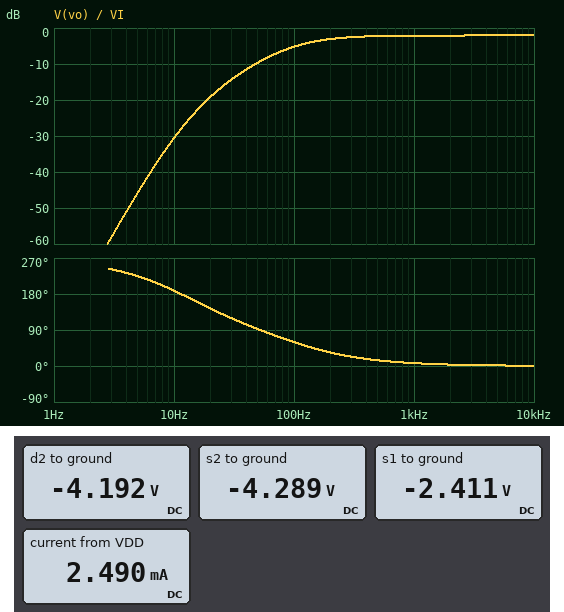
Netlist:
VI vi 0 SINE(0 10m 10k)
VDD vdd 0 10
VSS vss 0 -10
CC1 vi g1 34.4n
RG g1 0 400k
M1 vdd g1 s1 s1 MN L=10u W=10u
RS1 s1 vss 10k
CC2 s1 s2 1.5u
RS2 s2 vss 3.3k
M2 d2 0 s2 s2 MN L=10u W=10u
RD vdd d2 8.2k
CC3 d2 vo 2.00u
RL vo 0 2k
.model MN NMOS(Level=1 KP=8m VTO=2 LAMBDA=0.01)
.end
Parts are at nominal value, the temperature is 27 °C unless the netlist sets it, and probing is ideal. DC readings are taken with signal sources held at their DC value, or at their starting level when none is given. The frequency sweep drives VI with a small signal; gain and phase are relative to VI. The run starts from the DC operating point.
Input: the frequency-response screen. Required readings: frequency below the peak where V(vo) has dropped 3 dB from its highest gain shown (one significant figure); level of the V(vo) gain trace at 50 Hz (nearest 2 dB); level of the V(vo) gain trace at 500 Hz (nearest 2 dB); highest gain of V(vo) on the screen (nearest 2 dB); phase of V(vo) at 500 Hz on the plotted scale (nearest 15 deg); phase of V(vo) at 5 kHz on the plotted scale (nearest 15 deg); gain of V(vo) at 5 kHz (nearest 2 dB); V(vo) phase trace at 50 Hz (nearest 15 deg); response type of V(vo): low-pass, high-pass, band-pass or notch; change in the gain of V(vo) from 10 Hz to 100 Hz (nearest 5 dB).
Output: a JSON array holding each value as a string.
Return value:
["100 Hz", "-10 dB", "-2 dB", "-2 dB", "15 deg", "0 deg", "-2 dB", "90 deg", "high-pass", "25 dB"]
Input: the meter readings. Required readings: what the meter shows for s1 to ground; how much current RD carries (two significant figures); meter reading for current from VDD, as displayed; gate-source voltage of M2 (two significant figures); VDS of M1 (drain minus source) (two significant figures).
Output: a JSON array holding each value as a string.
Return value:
["-2.411 V", "1.7 mA", "2.490 mA", "4.3 V", "12 V"]
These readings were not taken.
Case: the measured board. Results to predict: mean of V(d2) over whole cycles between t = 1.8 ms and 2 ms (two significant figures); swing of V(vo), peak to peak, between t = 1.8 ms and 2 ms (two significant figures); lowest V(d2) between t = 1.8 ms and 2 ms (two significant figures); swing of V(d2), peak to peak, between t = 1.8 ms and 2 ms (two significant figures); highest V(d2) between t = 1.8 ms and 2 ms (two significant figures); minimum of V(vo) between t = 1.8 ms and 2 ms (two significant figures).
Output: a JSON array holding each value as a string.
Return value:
["-4.2 V", "16 mV", "-4.2 V", "16 mV", "-4.2 V", "-7.9 mV"]
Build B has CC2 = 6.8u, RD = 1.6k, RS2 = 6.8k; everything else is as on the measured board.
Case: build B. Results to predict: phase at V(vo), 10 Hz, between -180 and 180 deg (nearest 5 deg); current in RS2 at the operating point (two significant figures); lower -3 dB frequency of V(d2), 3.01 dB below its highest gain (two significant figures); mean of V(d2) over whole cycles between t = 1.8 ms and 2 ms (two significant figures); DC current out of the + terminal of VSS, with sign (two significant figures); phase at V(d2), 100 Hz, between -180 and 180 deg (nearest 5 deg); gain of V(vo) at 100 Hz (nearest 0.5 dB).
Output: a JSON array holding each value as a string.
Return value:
["-165 deg", "1.1 mA", "35 Hz", "8.2 V", "-1.9 mA", "25 deg", "3.5 dB"]
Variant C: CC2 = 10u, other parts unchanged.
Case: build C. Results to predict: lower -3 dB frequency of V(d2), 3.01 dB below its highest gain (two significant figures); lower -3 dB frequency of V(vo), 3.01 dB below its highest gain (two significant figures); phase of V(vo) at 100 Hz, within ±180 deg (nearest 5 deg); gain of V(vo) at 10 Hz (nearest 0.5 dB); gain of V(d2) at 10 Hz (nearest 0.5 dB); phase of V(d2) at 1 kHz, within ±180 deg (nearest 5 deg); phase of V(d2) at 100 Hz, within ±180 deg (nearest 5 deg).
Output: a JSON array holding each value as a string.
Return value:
["14 Hz", "45 Hz", "30 deg", "-19.5 dB", "-7.0 dB", "0 deg", "10 deg"]
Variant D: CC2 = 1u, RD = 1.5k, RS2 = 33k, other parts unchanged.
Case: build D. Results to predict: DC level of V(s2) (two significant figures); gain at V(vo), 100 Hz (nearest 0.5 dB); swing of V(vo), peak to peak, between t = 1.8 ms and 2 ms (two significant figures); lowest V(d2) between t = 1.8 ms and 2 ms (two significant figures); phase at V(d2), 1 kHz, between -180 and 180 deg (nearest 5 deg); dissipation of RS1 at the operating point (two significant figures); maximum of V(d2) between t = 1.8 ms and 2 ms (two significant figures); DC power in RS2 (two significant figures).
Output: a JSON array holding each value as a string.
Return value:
["-2.2 V", "-7.0 dB", "22 mV", "9.6 V", "10 deg", "5.8 mW", "9.7 V", "1.8 mW"]
